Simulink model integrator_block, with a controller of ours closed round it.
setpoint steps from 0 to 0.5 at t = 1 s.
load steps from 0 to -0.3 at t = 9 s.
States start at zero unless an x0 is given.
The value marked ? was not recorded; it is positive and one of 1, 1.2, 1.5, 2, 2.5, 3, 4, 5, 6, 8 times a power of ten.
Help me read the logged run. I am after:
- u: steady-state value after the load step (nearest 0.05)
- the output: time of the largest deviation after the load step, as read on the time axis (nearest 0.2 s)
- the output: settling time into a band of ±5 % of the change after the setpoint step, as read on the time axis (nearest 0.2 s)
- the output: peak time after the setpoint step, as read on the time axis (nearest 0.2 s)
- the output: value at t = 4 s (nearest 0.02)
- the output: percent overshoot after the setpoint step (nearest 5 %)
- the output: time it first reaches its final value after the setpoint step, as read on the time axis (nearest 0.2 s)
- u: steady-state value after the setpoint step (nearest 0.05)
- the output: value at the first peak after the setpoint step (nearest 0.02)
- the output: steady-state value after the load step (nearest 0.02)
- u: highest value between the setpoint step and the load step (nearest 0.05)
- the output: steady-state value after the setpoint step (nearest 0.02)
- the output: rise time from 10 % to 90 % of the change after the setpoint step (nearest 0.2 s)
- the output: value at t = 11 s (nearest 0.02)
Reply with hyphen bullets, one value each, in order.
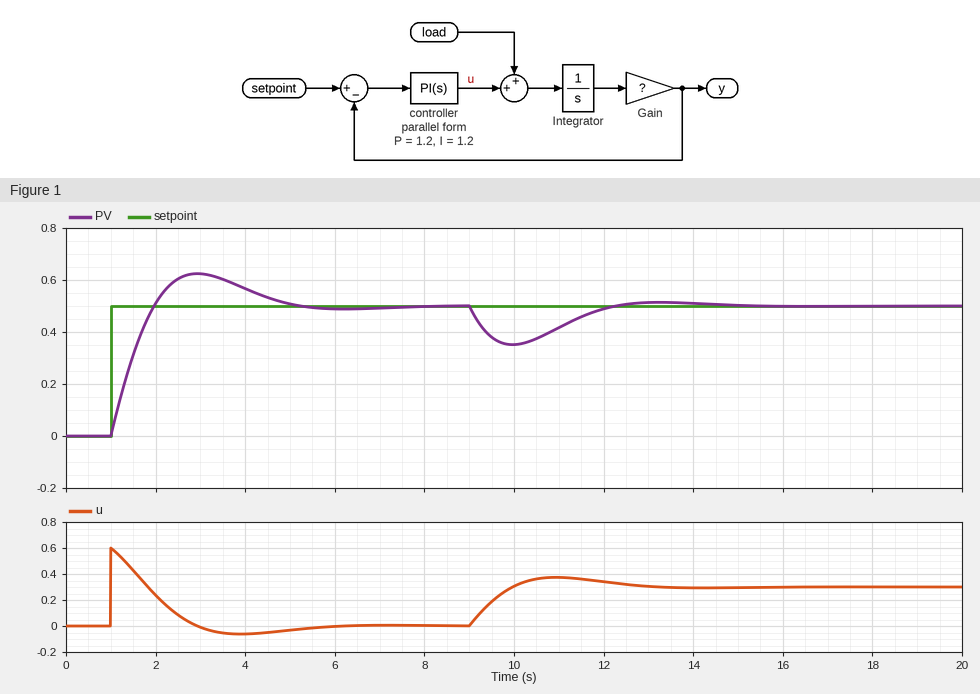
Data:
- 0.30
- 10.0 s
- 4.6 s
- 3.0 s
- 0.56
- 25 %
- 2.0 s
- 0.00
- 0.62
- 0.50
- 0.60
- 0.50
- 0.8 s
- 0.42
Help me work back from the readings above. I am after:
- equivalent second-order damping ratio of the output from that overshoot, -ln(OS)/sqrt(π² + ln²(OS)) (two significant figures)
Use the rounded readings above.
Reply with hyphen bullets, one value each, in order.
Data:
- 0.40
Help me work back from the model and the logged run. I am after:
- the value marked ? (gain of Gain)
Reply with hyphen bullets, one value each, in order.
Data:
- 1.2
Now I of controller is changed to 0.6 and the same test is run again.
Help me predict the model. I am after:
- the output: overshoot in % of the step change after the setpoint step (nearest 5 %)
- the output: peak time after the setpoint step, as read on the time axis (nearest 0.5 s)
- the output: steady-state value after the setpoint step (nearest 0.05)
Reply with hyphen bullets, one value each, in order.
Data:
- 15 %
- 3.5 s
- 0.50
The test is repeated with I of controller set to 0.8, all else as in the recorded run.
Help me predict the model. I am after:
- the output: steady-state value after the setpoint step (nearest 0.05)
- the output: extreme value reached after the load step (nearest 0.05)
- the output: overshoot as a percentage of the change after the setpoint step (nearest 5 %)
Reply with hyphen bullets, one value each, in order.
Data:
- 0.50
- 0.35
- 20 %
